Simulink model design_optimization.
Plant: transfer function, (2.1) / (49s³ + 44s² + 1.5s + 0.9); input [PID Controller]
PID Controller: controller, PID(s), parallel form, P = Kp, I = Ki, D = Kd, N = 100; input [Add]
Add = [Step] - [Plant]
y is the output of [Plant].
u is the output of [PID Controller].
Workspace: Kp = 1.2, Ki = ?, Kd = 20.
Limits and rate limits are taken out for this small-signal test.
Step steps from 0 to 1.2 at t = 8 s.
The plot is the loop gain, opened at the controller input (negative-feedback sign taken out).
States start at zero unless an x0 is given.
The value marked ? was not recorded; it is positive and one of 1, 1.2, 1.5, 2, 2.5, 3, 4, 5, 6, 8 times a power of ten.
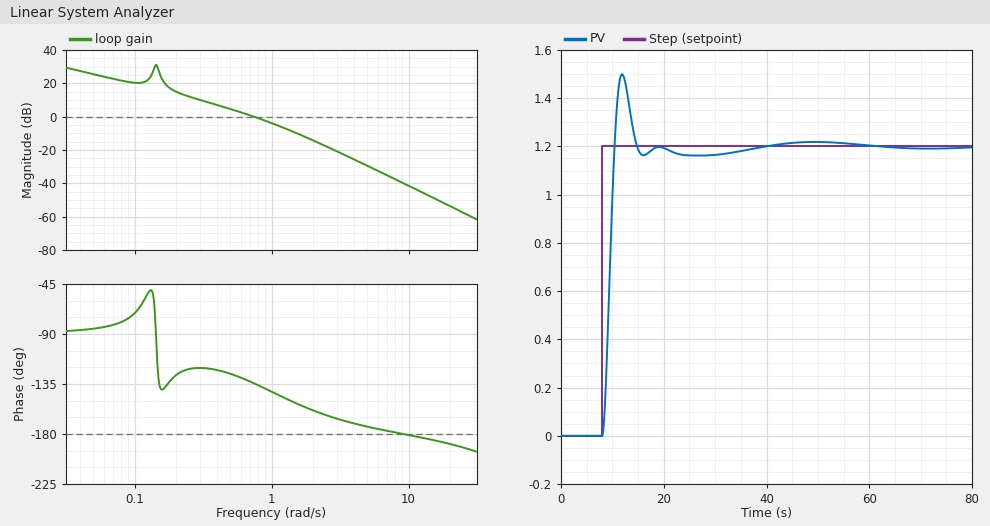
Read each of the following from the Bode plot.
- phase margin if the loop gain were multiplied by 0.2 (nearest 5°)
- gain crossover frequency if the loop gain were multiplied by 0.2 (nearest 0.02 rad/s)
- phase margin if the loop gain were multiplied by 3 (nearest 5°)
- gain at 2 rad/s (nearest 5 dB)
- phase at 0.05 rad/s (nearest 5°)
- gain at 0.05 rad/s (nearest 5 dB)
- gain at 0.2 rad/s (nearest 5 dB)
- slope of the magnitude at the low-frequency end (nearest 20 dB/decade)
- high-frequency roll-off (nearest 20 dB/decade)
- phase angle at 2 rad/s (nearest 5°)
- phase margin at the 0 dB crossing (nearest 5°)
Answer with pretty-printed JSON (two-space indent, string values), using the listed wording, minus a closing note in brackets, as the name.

{
  "phase margin if the loop gain were multiplied by 0.2": "55°",
  "gain crossover frequency if the loop gain were multiplied by 0.2": "0.22 rad/s",
  "phase margin if the loop gain were multiplied by 3": "30°",
  "gain at 2 rad/s": "-15 dB",
  "phase at 0.05 rad/s": "-85°",
  "gain at 0.05 rad/s": "25 dB",
  "gain at 0.2 rad/s": "15 dB",
  "slope of the magnitude at the low-frequency end": "-20 dB/decade",
  "high-frequency roll-off": "-40 dB/decade",
  "phase angle at 2 rad/s": "-160°",
  "phase margin at the 0 dB crossing": "45°"
}
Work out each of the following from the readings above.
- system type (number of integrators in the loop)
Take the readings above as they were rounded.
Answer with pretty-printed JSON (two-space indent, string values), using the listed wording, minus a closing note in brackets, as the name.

{
  "system type": "1"
}
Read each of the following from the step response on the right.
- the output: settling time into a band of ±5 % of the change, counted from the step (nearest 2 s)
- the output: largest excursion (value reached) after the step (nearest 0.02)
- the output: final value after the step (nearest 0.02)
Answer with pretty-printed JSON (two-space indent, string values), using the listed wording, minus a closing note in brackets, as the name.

{
  "the output: settling time into a band of ±5 % of the change, counted from the step": "6 s",
  "the output: largest excursion (value reached) after the step": "1.50",
  "the output: final value after the step": "1.20"
}
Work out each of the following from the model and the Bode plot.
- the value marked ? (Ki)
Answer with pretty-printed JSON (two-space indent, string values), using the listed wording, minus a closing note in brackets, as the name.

{
  "the value marked ?": "0.4"
}
